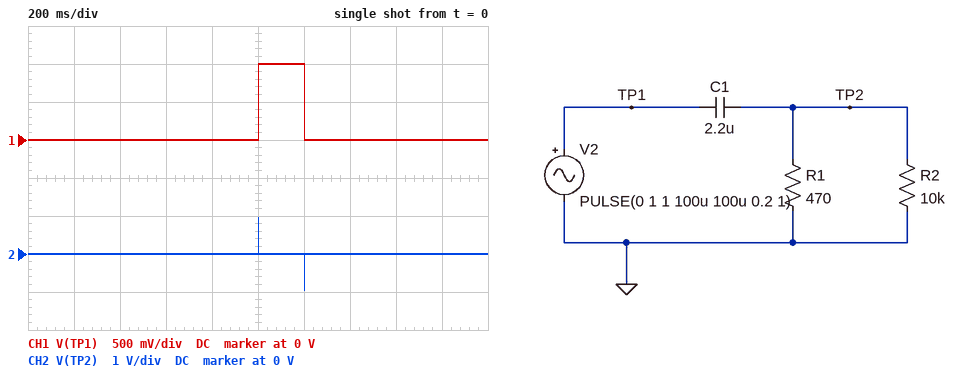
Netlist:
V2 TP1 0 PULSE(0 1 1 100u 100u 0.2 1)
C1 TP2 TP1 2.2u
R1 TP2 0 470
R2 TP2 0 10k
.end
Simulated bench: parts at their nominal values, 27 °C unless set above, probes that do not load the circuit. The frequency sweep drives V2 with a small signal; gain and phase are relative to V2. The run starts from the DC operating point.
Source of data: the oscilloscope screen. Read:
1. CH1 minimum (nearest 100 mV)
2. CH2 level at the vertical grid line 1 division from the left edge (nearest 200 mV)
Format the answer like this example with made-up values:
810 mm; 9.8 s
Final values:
0 V; 0 V
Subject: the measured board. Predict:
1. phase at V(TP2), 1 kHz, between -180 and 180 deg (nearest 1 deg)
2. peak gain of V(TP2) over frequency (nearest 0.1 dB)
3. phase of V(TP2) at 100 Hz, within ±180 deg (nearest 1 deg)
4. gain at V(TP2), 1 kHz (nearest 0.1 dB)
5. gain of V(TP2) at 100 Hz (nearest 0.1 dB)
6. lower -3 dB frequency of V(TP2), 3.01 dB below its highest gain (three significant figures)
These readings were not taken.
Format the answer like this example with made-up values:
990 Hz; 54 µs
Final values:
9 deg; 0 dB; 58 deg; -0.1 dB; -5.6 dB; 161 Hz
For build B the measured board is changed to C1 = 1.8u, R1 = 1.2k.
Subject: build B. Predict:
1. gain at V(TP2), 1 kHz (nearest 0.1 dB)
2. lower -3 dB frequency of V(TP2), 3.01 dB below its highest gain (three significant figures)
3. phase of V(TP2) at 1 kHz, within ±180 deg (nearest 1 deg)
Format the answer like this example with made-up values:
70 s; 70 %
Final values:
0 dB; 82.5 Hz; 5 deg
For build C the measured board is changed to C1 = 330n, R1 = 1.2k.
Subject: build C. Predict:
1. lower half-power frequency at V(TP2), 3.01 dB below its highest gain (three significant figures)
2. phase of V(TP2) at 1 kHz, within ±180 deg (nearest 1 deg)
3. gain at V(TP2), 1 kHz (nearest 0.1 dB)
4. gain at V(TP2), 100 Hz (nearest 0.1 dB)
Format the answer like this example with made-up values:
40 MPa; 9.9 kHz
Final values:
450 Hz; 24 deg; -0.8 dB; -13.3 dB
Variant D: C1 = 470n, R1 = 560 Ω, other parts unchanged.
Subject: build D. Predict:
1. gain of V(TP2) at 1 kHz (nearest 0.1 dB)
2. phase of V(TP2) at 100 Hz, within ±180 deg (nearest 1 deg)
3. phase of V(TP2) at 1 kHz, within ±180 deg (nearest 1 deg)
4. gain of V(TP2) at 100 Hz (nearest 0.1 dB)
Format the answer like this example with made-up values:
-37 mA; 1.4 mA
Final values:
-1.5 dB; 81 deg; 33 deg; -16.2 dB
